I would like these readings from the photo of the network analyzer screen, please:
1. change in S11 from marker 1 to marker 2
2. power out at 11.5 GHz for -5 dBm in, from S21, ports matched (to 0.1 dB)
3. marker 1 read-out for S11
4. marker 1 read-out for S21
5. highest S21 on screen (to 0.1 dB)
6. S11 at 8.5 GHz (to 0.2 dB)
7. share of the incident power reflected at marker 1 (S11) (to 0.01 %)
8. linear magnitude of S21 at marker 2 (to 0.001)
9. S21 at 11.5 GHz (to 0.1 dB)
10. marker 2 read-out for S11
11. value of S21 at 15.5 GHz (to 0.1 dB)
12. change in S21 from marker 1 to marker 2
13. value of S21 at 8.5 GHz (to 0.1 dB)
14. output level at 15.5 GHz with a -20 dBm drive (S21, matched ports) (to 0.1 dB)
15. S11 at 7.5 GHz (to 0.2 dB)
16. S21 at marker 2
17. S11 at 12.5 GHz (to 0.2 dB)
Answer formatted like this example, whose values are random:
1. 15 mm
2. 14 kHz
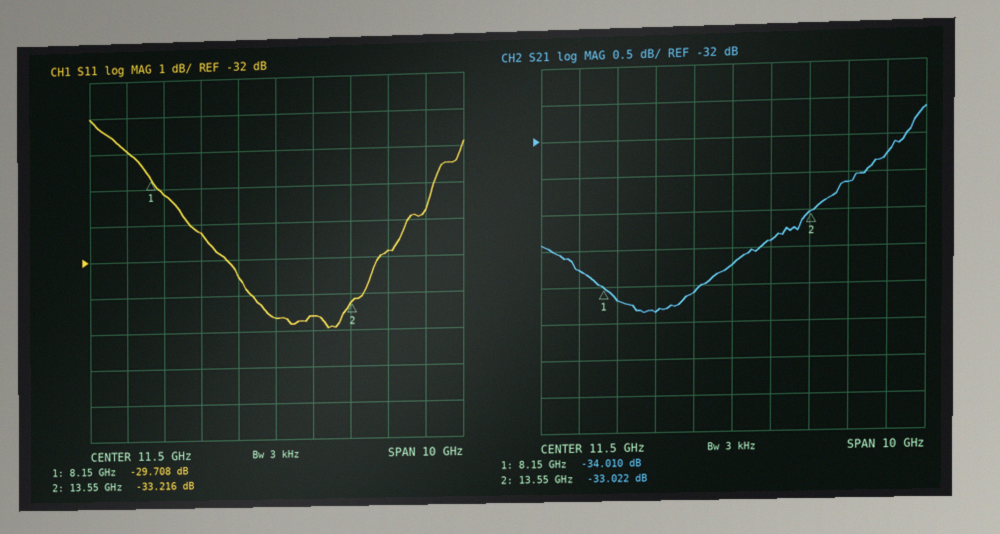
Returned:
1. -3.508 dB
2. -38.7 dBm
3. -29.708 dB
4. -34.010 dB
5. -31.6 dB
6. -30.2 dB
7. 0.11 %
8. 0.022
9. -33.7 dB
10. -33.216 dB
11. -32.3 dB
12. 0.988 dB
13. -34.2 dB
14. -52.3 dBm
15. -29.0 dB
16. -33.022 dB
17. -33.6 dB
